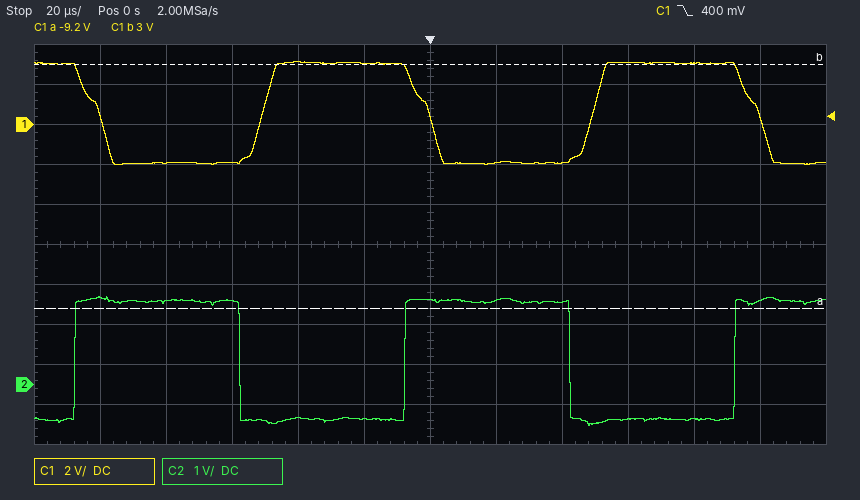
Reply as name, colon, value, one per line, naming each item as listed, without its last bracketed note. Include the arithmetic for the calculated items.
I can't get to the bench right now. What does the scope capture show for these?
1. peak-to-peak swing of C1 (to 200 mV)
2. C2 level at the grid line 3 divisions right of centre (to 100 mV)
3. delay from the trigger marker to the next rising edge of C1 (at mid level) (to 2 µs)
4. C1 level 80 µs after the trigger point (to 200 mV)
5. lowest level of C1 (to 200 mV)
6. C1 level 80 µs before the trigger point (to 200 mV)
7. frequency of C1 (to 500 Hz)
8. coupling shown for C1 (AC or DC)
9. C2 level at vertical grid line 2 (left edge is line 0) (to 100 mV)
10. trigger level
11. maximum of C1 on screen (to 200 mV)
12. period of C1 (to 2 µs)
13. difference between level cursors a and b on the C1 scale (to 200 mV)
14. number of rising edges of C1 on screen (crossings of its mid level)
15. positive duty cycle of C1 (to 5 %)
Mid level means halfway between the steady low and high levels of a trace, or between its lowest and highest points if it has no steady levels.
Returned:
peak-to-peak swing of C1: 3.2 V − (-2.0 V) = 5.2 V
C2 level at the grid line 3 divisions right of centre: -900 mV
delay from the trigger marker to the next rising edge of C1 (at mid level): 50 µs
C1 level 80 µs after the trigger point: 3.0 V
lowest level of C1: -2.0 V
C1 level 80 µs before the trigger point: -2.0 V
frequency of C1: 1 / 100 µs ≈ 10.0 kHz
coupling shown for C1: DC
C2 level at vertical grid line 2 (left edge is line 0): 2.1 V
trigger level: 400 mV
maximum of C1 on screen: 3.2 V
period of C1: 100 µs
difference between level cursors a and b on the C1 scale: 12.2 V
number of rising edges of C1 on screen: 2
positive duty cycle of C1: 50 %
